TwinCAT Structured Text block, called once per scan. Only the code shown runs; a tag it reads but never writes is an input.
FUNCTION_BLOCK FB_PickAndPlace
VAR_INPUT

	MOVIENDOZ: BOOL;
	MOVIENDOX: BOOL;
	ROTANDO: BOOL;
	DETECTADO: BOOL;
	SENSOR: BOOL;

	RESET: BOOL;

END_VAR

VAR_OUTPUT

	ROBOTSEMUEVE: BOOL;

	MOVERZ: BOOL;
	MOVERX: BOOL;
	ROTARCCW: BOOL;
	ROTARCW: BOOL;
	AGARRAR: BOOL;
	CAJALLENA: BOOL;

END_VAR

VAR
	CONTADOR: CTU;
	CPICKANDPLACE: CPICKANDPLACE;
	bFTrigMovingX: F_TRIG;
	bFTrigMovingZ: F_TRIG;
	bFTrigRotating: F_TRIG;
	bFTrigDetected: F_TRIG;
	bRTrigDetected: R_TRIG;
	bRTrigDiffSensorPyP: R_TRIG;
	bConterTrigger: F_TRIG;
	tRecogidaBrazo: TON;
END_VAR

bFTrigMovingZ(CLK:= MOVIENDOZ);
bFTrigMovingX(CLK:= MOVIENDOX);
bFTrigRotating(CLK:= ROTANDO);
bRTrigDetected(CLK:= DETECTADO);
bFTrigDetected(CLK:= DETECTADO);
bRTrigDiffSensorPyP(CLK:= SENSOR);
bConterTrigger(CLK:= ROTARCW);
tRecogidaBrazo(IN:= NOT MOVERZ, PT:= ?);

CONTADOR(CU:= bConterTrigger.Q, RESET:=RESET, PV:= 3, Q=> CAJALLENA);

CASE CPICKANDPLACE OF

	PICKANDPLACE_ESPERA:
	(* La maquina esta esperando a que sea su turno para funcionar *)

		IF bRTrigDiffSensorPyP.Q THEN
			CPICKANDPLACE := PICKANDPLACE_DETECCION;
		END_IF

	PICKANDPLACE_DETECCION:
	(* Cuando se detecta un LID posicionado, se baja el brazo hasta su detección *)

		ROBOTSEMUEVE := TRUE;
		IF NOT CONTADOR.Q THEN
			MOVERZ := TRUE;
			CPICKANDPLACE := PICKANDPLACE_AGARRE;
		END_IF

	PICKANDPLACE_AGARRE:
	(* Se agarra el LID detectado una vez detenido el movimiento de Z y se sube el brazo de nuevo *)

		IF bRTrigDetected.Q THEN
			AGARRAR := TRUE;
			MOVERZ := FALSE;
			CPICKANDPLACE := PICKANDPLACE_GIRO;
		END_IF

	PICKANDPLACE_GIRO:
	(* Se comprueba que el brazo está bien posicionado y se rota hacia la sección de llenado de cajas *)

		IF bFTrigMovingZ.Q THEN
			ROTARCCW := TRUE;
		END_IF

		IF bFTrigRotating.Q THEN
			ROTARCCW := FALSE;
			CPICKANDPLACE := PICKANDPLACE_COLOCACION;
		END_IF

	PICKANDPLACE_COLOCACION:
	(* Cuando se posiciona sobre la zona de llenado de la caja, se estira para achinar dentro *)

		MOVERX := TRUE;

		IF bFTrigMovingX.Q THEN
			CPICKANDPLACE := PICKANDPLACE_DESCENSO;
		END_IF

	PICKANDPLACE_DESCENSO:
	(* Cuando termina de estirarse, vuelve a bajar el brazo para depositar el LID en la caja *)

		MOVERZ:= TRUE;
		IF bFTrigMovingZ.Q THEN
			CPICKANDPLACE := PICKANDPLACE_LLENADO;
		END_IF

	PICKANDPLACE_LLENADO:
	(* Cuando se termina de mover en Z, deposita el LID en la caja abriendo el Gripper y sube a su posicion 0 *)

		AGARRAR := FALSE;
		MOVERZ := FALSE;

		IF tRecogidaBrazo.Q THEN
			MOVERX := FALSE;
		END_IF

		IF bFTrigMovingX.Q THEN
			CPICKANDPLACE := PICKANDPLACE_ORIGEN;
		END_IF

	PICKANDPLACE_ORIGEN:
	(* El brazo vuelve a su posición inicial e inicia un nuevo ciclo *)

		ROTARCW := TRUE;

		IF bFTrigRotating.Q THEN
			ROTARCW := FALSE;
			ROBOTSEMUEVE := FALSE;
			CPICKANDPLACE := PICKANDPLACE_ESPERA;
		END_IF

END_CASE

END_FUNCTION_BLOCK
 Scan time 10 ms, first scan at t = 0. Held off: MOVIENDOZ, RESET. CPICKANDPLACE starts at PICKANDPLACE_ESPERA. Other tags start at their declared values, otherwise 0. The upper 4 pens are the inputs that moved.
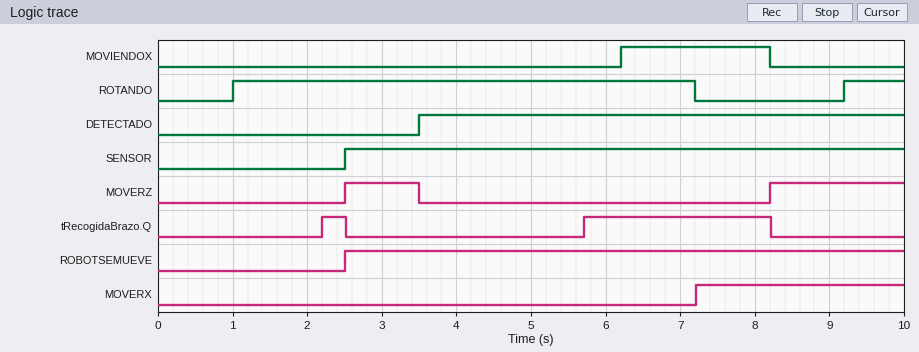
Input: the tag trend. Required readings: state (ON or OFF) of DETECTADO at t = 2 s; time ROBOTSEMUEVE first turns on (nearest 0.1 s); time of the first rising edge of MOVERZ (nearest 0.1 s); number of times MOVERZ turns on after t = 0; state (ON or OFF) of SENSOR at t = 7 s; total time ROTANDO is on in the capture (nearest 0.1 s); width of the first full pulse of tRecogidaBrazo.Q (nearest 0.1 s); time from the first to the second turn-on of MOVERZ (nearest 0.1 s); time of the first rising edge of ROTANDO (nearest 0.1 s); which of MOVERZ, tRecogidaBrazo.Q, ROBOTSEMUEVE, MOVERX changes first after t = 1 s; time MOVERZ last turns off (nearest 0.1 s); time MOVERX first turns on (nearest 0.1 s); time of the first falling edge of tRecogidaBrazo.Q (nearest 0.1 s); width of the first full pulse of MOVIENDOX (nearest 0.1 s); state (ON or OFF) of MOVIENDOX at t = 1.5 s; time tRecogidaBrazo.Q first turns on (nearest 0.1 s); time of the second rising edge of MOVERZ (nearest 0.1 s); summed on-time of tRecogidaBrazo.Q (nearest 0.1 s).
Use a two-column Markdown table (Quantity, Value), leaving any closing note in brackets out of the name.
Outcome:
| Quantity | Value |
|---|---|
| state (ON or OFF) of DETECTADO at t = 2 s | OFF |
| time ROBOTSEMUEVE first turns on | 2.5 s |
| time of the first rising edge of MOVERZ | 2.5 s |
| number of times MOVERZ turns on after t = 0 | 2 |
| state (ON or OFF) of SENSOR at t = 7 s | ON |
| total time ROTANDO is on in the capture | 7.0 s |
| width of the first full pulse of tRecogidaBrazo.Q | 0.3 s |
| time from the first to the second turn-on of MOVERZ | 5.7 s |
| time of the first rising edge of ROTANDO | 1.0 s |
| which of MOVERZ, tRecogidaBrazo.Q, ROBOTSEMUEVE, MOVERX changes first after t = 1 s | tRecogidaBrazo.Q |
| time MOVERZ last turns off | 3.5 s |
| time MOVERX first turns on | 7.2 s |
| time of the first falling edge of tRecogidaBrazo.Q | 2.5 s |
| width of the first full pulse of MOVIENDOX | 2.0 s |
| state (ON or OFF) of MOVIENDOX at t = 1.5 s | OFF |
| time tRecogidaBrazo.Q first turns on | 2.2 s |
| time of the second rising edge of MOVERZ | 8.2 s |
| summed on-time of tRecogidaBrazo.Q | 2.8 s |
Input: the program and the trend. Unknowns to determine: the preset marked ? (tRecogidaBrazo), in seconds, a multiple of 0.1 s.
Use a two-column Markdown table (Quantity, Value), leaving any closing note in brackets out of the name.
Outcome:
| Quantity | Value |
|---|---|
| the preset marked ? (tRecogidaBrazo), in seconds, a multiple of 0.1 s | 2.2 s |
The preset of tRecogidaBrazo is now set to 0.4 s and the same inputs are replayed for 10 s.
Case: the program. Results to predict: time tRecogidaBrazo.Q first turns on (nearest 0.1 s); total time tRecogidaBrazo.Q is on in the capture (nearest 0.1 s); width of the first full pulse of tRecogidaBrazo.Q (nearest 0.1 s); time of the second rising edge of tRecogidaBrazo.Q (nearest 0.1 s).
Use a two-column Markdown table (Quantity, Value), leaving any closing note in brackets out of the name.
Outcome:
| Quantity | Value |
|---|---|
| time tRecogidaBrazo.Q first turns on | 0.4 s |
| total time tRecogidaBrazo.Q is on in the capture | 6.4 s |
| width of the first full pulse of tRecogidaBrazo.Q | 2.1 s |
| time of the second rising edge of tRecogidaBrazo.Q | 3.9 s |
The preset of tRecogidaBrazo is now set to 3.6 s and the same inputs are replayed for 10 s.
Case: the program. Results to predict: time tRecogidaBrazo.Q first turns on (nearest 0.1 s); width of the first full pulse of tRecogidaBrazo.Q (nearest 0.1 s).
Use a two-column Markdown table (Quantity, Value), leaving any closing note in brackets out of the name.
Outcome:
| Quantity | Value |
|---|---|
| time tRecogidaBrazo.Q first turns on | 7.1 s |
| width of the first full pulse of tRecogidaBrazo.Q | 1.1 s |
